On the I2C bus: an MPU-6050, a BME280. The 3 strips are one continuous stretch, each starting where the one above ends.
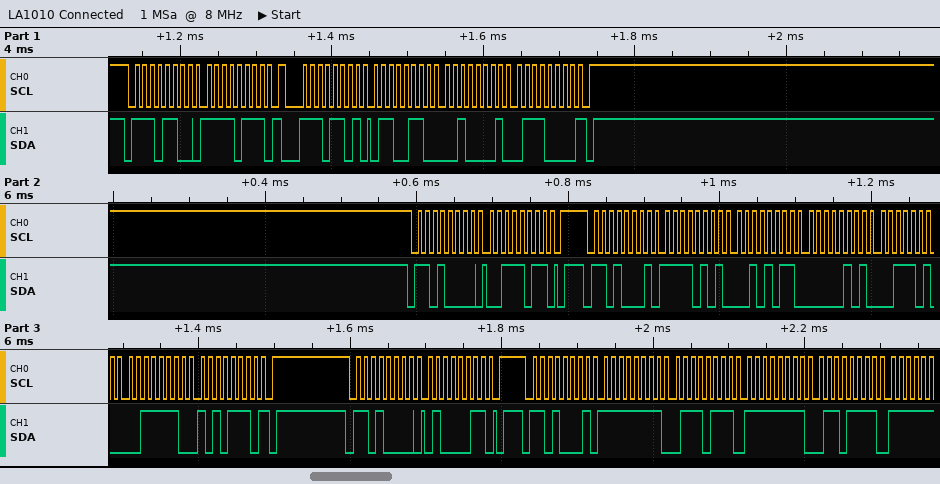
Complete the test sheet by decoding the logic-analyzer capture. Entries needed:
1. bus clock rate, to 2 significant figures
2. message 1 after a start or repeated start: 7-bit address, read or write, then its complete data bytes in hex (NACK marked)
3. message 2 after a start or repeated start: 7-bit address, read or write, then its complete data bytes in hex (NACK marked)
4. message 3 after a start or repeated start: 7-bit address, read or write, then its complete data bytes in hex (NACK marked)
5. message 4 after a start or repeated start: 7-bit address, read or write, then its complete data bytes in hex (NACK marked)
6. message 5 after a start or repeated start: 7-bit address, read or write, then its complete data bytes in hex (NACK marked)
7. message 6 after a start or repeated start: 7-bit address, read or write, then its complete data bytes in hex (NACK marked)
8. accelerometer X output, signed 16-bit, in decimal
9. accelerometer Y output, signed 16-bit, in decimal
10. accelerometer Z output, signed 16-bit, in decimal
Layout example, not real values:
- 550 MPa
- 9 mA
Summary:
- 100 kHz
- 0x76 write: F7
- 0x76 read: 66 21 70 NACK
- 0x68 write: 3B
- 0x68 read: F5 2B 05 3A 3E AE NACK
- 0x68 write: 43
- 0x68 read: FF 77 FF 6F
- -2773
- 1338
- 16046
